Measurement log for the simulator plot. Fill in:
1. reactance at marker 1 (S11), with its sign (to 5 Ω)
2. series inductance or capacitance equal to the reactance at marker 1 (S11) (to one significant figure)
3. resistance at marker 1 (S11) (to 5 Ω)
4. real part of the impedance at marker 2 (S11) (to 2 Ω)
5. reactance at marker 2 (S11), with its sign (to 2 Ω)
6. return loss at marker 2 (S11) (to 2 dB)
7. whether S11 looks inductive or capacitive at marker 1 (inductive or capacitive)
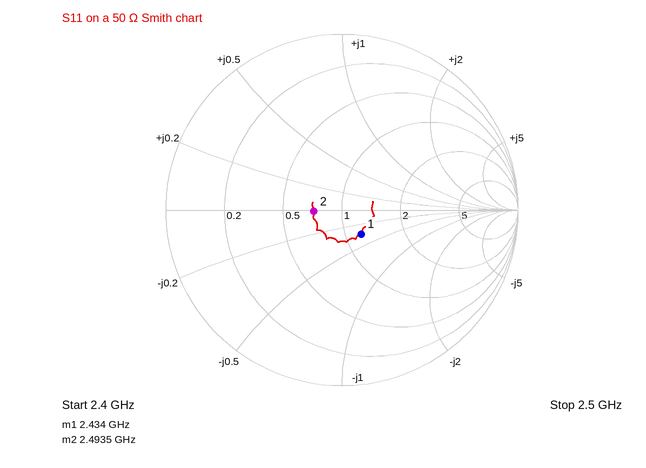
-15 Ω
4 pF
60 Ω
36 Ω
0 Ω
16 dB
capacitive
